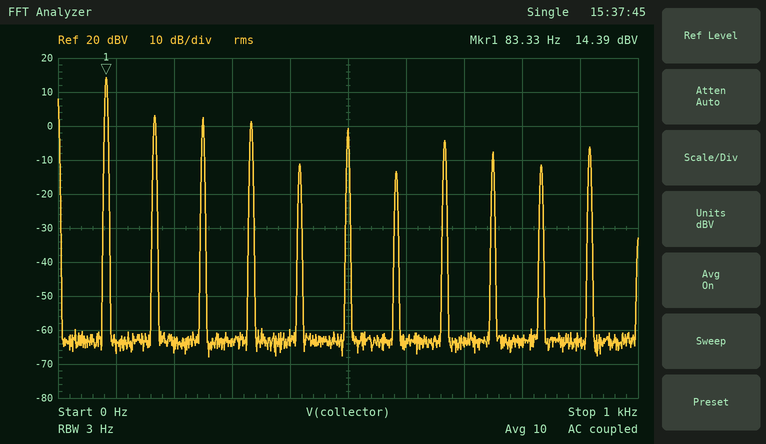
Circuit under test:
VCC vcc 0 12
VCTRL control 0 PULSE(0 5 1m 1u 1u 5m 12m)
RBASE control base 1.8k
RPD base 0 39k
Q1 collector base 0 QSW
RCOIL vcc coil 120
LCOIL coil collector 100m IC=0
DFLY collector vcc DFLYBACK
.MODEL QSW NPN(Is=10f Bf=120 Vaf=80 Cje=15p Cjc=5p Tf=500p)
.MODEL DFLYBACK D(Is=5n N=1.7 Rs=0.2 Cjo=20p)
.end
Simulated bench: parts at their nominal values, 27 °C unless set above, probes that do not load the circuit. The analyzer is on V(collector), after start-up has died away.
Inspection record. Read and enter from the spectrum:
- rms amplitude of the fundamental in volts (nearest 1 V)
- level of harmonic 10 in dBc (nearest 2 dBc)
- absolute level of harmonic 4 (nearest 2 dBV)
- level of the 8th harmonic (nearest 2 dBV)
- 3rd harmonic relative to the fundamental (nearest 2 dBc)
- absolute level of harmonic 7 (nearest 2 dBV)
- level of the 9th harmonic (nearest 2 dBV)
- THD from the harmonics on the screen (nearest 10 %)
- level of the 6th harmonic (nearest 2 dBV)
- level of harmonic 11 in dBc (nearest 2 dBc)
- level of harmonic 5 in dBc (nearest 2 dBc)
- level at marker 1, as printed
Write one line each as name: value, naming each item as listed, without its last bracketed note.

rms amplitude of the fundamental in volts: 5 V
level of harmonic 10 in dBc: -26 dBc
absolute level of harmonic 4: 2 dBV
level of the 8th harmonic: -4 dBV
3rd harmonic relative to the fundamental: -12 dBc
absolute level of harmonic 7: -14 dBV
level of the 9th harmonic: -8 dBV
THD from the harmonics on the screen: 50 %
level of the 6th harmonic: 0 dBV
level of harmonic 11 in dBc: -20 dBc
level of harmonic 5 in dBc: -26 dBc
level at marker 1, as printed: 14.39 dBV
